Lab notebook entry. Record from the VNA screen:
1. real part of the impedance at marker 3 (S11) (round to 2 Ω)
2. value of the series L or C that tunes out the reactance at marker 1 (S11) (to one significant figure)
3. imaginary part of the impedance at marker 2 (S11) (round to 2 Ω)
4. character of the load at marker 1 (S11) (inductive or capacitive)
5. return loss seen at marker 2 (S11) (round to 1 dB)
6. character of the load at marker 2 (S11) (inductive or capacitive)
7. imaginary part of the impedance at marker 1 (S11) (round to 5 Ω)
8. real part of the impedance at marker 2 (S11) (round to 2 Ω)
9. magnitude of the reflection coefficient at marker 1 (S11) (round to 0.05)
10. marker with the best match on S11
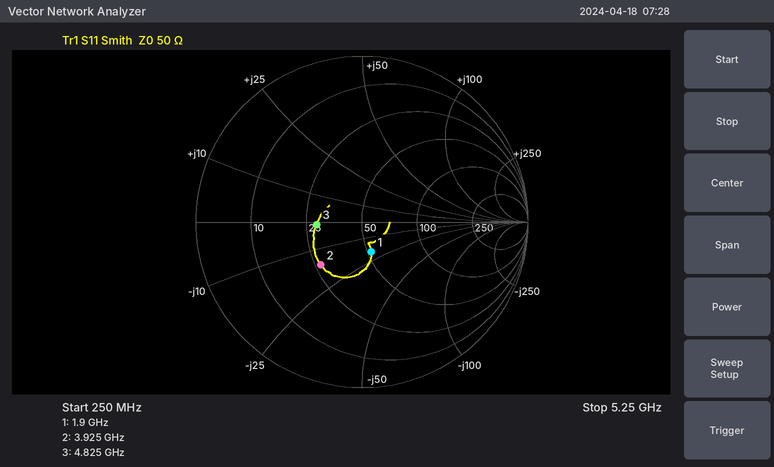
28 Ω
2 nH
-16 Ω
capacitive
9 dB
capacitive
-20 Ω
26 Ω
0.20
marker 1
